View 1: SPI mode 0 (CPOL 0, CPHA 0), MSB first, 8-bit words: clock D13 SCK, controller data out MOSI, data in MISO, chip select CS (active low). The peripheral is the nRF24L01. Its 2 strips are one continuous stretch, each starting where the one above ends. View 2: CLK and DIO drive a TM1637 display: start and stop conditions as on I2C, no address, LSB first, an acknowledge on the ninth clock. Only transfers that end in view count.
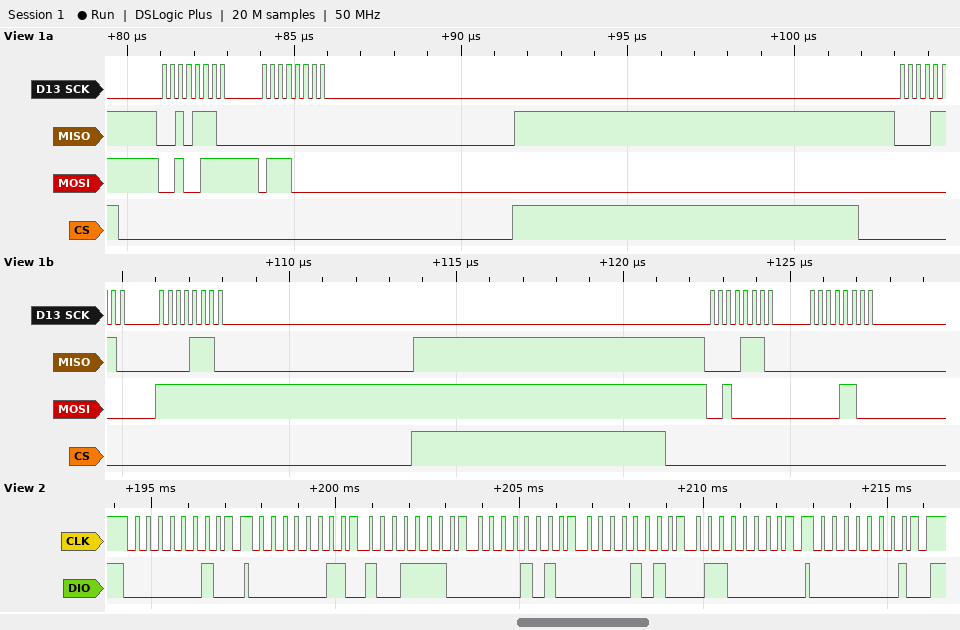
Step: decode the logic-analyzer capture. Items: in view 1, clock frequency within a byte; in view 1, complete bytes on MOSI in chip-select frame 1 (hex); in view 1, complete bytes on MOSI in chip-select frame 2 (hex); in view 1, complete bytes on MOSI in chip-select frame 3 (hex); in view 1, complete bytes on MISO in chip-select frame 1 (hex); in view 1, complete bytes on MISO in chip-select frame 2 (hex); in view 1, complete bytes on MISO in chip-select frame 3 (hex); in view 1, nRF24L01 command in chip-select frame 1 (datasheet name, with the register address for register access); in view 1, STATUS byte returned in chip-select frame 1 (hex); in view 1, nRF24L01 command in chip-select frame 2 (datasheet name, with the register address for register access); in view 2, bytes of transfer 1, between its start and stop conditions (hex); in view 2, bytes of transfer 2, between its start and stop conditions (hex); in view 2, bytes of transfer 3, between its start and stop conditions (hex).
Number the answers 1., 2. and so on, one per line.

1. 4 MHz
2. 27 70
3. 00 FF
4. 20 0C
5. 2E 00
6. 0E 0E
7. 0E 00
8. W_REGISTER 0x07
9. 0x2E
10. R_REGISTER 0x00
11. 40
12. C0 79 50 50 06
13. 80
